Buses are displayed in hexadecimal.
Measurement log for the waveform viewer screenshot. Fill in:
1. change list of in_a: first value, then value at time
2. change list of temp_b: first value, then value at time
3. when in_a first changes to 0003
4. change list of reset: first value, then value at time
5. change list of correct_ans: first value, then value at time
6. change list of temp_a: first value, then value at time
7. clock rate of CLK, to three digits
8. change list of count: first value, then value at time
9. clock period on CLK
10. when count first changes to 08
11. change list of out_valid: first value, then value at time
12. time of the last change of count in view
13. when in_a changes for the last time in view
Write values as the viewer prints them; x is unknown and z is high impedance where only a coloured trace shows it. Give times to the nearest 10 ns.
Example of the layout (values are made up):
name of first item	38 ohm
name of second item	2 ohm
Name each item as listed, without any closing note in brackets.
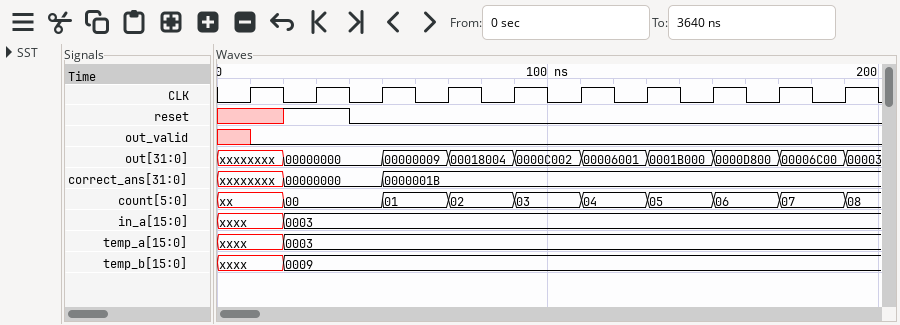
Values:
change list of in_a: first value, then value at time	xxxx, 0003 at 20 ns
change list of temp_b: first value, then value at time	xxxx, 0009 at 20 ns
when in_a first changes to 0003	20 ns
change list of reset: first value, then value at time	x, 1 at 20 ns, 0 at 40 ns
change list of correct_ans: first value, then value at time	xxxxxxxx, 00000000 at 20 ns, 0000001B at 50 ns
change list of temp_a: first value, then value at time	xxxx, 0003 at 20 ns
clock rate of CLK, to three digits	50.0 MHz
change list of count: first value, then value at time	xx, 00 at 20 ns, 01 at 50 ns, 02 at 70 ns, 03 at 90 ns, 04 at 110 ns, 05 at 130 ns, 06 at 150 ns, 07 at 170 ns, 08 at 190 ns
clock period on CLK	20 ns
when count first changes to 08	190 ns
change list of out_valid: first value, then value at time	x, 0 at 10 ns
time of the last change of count in view	190 ns
when in_a changes for the last time in view	20 ns
